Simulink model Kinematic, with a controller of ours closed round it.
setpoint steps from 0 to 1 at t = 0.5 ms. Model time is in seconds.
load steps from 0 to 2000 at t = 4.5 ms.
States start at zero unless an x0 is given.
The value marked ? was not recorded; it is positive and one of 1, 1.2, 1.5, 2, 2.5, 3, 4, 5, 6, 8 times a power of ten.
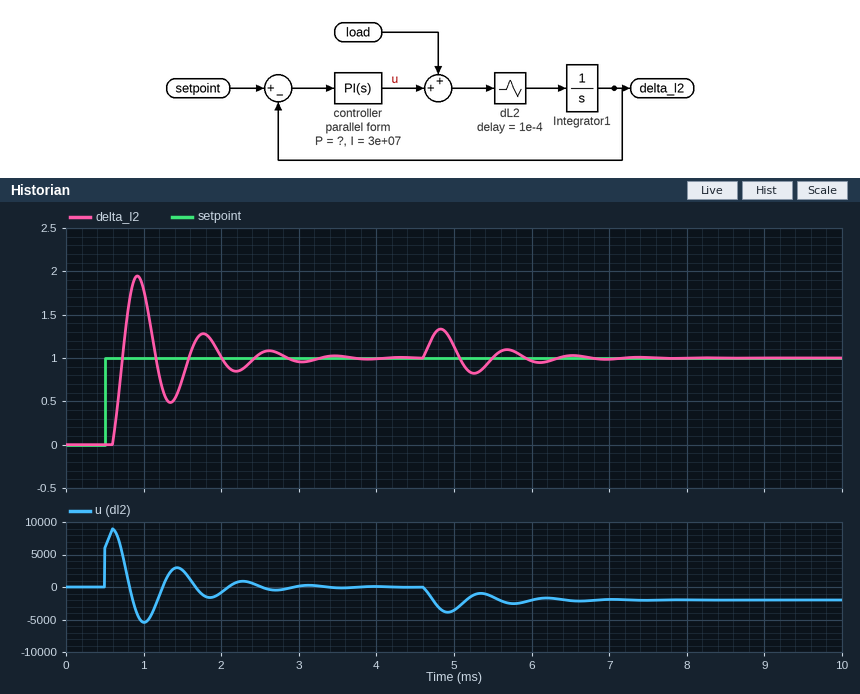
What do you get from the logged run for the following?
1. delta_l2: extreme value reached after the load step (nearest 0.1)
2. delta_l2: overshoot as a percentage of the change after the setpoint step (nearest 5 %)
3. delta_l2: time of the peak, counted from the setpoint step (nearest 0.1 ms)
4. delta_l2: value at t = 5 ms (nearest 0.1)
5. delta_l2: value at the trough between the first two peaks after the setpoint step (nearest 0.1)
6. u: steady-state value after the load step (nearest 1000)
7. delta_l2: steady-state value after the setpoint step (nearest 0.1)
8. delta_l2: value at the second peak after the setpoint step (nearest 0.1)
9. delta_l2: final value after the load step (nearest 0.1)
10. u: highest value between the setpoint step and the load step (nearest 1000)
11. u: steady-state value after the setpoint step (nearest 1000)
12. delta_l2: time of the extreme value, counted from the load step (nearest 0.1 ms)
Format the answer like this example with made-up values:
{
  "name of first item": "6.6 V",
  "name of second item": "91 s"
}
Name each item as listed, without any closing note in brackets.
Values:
{
  "delta_l2: extreme value reached after the load step": "1.3",
  "delta_l2: overshoot as a percentage of the change after the setpoint step": "95 %",
  "delta_l2: time of the peak, counted from the setpoint step": "0.4 ms",
  "delta_l2: value at t = 5 ms": "1.1",
  "delta_l2: value at the trough between the first two peaks after the setpoint step": "0.5",
  "u: steady-state value after the load step": "-2000",
  "delta_l2: steady-state value after the setpoint step": "1.0",
  "delta_l2: value at the second peak after the setpoint step": "1.3",
  "delta_l2: final value after the load step": "1.0",
  "u: highest value between the setpoint step and the load step": "9000",
  "u: steady-state value after the setpoint step": "0",
  "delta_l2: time of the extreme value, counted from the load step": "0.3 ms"
}
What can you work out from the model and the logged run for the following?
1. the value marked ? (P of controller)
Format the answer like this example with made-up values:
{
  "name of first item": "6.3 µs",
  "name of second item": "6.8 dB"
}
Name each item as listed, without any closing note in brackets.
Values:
{
  "the value marked ?": "6000"
}
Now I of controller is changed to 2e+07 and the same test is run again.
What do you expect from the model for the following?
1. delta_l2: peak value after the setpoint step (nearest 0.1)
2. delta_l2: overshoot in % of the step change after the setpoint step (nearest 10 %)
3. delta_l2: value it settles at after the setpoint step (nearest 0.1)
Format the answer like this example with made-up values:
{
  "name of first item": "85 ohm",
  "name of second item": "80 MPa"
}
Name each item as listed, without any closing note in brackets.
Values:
{
  "delta_l2: peak value after the setpoint step": "1.7",
  "delta_l2: overshoot in % of the step change after the setpoint step": "70 %",
  "delta_l2: value it settles at after the setpoint step": "1.0"
}
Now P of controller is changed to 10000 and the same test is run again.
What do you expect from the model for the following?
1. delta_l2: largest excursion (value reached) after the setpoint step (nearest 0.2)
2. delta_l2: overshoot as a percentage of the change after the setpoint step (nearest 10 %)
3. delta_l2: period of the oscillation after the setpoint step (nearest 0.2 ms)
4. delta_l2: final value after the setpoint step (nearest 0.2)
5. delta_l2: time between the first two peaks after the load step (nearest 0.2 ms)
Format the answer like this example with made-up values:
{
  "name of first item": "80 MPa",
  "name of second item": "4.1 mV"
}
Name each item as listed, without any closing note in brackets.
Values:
{
  "delta_l2: largest excursion (value reached) after the setpoint step": "2.0",
  "delta_l2: overshoot as a percentage of the change after the setpoint step": "100 %",
  "delta_l2: period of the oscillation after the setpoint step": "0.6 ms",
  "delta_l2: final value after the setpoint step": "1.0",
  "delta_l2: time between the first two peaks after the load step": "0.6 ms"
}
